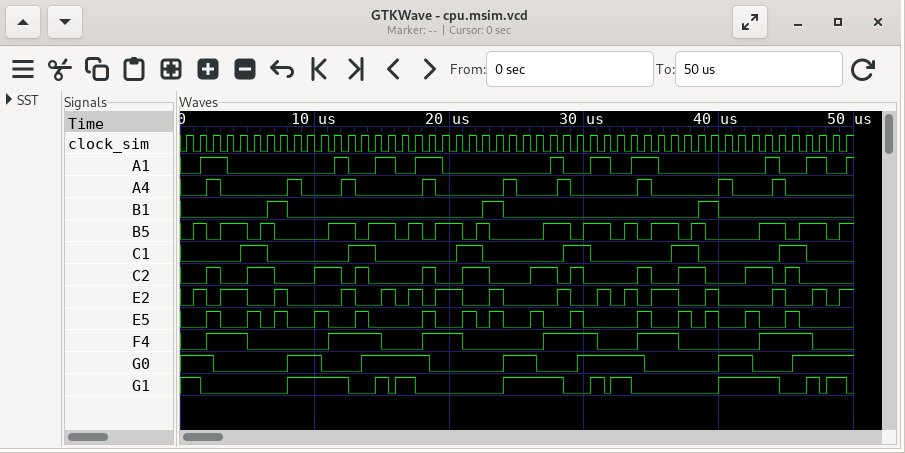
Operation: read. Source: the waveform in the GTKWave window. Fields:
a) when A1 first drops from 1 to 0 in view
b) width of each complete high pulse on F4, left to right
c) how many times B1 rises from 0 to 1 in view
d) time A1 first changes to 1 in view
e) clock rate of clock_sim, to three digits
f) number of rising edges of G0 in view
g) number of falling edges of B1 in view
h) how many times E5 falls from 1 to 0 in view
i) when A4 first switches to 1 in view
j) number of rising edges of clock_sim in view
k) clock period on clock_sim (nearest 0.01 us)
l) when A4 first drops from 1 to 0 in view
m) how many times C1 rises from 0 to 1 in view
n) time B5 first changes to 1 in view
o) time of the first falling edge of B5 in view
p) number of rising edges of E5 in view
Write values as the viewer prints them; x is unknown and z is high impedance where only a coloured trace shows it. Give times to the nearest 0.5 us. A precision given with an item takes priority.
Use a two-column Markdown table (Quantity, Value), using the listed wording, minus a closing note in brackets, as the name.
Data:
| Quantity | Value |
|---|---|
| when A1 first drops from 1 to 0 in view | 3.5 us |
| width of each complete high pulse on F4, left to right | 3 us, 4 us, 3 us, 4 us, 3 us, 4 us |
| how many times B1 rises from 0 to 1 in view | 3 |
| time A1 first changes to 1 in view | 1.5 us |
| clock rate of clock_sim, to three digits | 1.00 MHz |
| number of rising edges of G0 in view | 6 |
| number of falling edges of B1 in view | 3 |
| how many times E5 falls from 1 to 0 in view | 15 |
| when A4 first switches to 1 in view | 2 us |
| number of rising edges of clock_sim in view | 50 |
| clock period on clock_sim | 1 us |
| when A4 first drops from 1 to 0 in view | 3 us |
| how many times C1 rises from 0 to 1 in view | 6 |
| time B5 first changes to 1 in view | 1 us |
| time of the first falling edge of B5 in view | 2 us |
| number of rising edges of E5 in view | 15 |
